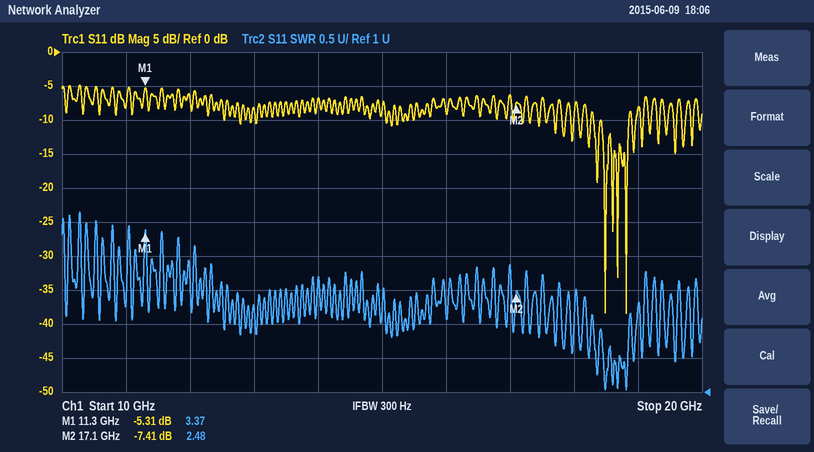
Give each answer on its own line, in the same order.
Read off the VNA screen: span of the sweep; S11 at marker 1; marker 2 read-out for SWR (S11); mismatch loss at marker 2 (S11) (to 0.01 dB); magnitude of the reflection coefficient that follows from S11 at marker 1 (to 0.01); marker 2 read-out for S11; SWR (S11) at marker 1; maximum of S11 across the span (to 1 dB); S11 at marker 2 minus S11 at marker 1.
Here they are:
10 GHz
-5.31 dB
2.48
0.87 dB
0.54
-7.41 dB
3.37
-5 dB
-2.10 dB
